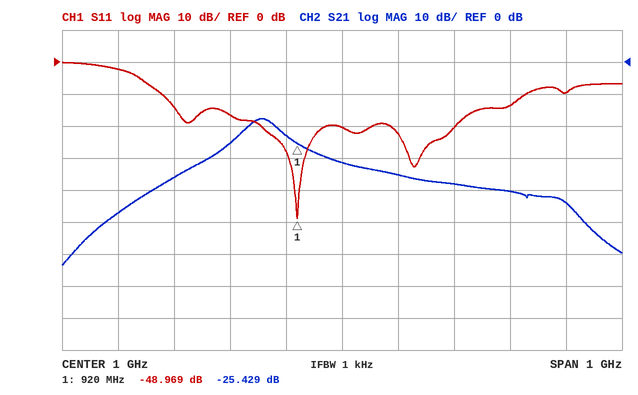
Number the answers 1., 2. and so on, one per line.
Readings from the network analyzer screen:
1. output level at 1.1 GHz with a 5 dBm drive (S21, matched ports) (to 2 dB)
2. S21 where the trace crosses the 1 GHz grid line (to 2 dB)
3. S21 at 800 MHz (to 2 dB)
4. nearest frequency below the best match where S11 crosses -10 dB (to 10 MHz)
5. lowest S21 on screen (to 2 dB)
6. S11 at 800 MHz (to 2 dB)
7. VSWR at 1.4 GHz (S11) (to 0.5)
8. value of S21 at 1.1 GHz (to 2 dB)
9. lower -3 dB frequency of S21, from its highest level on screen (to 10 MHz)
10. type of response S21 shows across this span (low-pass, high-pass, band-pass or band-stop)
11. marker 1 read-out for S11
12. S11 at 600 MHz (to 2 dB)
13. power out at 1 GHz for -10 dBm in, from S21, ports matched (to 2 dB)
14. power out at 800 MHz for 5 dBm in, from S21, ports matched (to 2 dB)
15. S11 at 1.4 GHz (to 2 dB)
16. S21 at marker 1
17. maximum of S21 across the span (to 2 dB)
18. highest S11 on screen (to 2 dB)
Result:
1. -30 dBm
2. -32 dB
3. -26 dB
4. 680 MHz
5. -64 dB
6. -16 dB
7. 2.0
8. -36 dB
9. 830 MHz
10. band-pass
11. -48.969 dB
12. -2 dB
13. -42 dBm
14. -20 dBm
15. -10 dB
16. -25.429 dB
17. -18 dB
18. 0 dB
